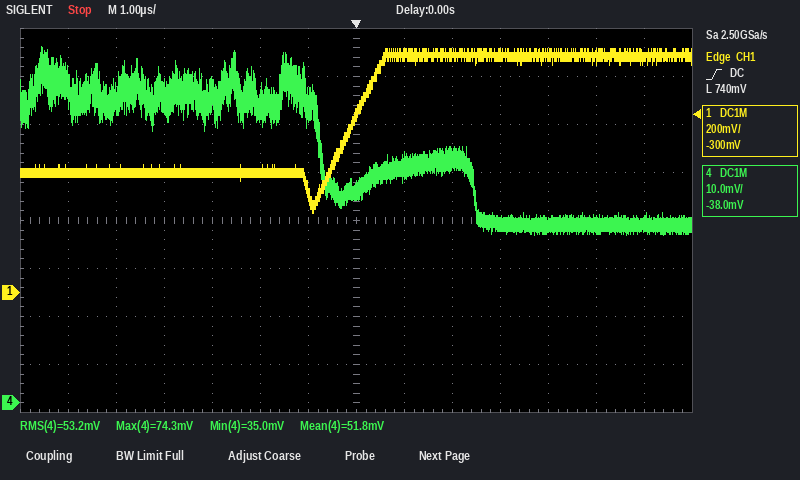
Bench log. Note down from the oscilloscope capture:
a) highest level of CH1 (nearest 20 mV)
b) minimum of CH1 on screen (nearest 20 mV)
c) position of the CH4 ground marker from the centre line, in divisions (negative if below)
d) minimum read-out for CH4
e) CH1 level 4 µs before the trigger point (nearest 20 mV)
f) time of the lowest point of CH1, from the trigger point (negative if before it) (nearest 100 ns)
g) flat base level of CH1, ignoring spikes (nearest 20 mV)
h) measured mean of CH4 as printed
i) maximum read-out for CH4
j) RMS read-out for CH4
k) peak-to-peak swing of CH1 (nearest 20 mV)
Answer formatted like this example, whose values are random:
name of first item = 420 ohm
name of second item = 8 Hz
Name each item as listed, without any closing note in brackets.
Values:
highest level of CH1 = 1.02 V
minimum of CH1 on screen = 340 mV
position of the CH4 ground marker from the centre line, in divisions = -3.8 div
minimum read-out for CH4 = 35.0 mV
CH1 level 4 µs before the trigger point = 500 mV
time of the lowest point of CH1, from the trigger point (negative if before it) = -900 ns
flat base level of CH1, ignoring spikes = 500 mV
measured mean of CH4 as printed = 51.8 mV
maximum read-out for CH4 = 74.3 mV
RMS read-out for CH4 = 53.2 mV
peak-to-peak swing of CH1 = 680 mV
